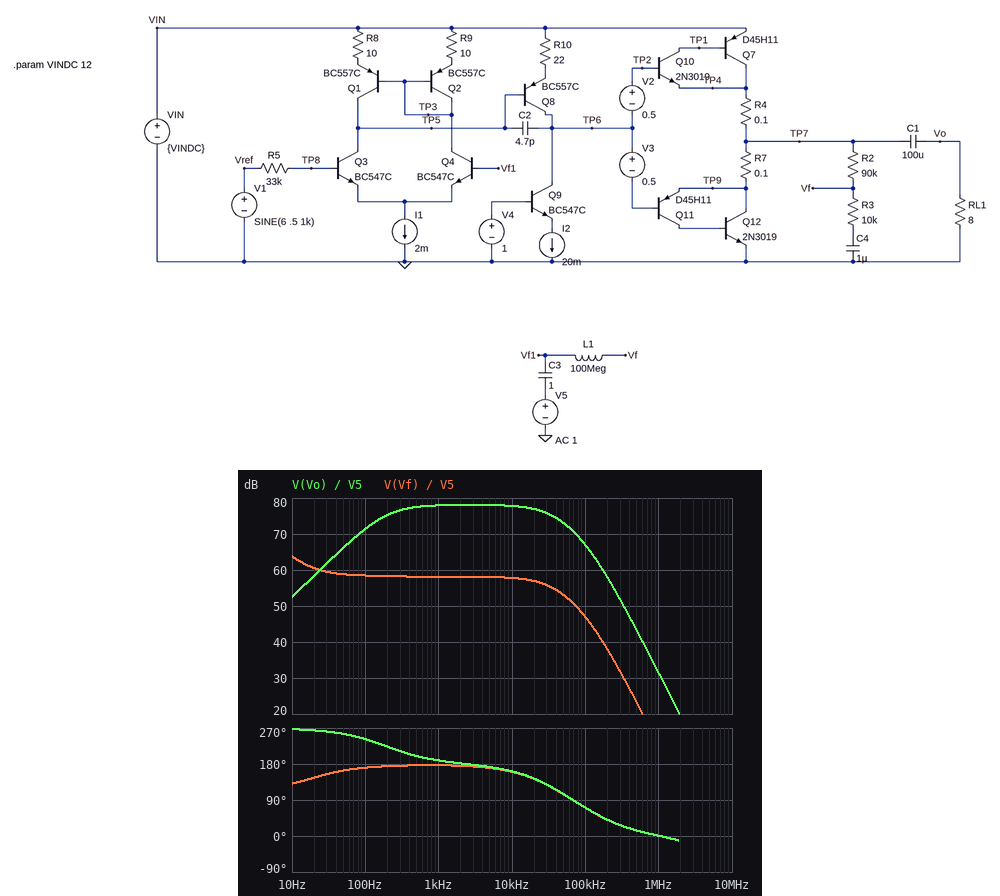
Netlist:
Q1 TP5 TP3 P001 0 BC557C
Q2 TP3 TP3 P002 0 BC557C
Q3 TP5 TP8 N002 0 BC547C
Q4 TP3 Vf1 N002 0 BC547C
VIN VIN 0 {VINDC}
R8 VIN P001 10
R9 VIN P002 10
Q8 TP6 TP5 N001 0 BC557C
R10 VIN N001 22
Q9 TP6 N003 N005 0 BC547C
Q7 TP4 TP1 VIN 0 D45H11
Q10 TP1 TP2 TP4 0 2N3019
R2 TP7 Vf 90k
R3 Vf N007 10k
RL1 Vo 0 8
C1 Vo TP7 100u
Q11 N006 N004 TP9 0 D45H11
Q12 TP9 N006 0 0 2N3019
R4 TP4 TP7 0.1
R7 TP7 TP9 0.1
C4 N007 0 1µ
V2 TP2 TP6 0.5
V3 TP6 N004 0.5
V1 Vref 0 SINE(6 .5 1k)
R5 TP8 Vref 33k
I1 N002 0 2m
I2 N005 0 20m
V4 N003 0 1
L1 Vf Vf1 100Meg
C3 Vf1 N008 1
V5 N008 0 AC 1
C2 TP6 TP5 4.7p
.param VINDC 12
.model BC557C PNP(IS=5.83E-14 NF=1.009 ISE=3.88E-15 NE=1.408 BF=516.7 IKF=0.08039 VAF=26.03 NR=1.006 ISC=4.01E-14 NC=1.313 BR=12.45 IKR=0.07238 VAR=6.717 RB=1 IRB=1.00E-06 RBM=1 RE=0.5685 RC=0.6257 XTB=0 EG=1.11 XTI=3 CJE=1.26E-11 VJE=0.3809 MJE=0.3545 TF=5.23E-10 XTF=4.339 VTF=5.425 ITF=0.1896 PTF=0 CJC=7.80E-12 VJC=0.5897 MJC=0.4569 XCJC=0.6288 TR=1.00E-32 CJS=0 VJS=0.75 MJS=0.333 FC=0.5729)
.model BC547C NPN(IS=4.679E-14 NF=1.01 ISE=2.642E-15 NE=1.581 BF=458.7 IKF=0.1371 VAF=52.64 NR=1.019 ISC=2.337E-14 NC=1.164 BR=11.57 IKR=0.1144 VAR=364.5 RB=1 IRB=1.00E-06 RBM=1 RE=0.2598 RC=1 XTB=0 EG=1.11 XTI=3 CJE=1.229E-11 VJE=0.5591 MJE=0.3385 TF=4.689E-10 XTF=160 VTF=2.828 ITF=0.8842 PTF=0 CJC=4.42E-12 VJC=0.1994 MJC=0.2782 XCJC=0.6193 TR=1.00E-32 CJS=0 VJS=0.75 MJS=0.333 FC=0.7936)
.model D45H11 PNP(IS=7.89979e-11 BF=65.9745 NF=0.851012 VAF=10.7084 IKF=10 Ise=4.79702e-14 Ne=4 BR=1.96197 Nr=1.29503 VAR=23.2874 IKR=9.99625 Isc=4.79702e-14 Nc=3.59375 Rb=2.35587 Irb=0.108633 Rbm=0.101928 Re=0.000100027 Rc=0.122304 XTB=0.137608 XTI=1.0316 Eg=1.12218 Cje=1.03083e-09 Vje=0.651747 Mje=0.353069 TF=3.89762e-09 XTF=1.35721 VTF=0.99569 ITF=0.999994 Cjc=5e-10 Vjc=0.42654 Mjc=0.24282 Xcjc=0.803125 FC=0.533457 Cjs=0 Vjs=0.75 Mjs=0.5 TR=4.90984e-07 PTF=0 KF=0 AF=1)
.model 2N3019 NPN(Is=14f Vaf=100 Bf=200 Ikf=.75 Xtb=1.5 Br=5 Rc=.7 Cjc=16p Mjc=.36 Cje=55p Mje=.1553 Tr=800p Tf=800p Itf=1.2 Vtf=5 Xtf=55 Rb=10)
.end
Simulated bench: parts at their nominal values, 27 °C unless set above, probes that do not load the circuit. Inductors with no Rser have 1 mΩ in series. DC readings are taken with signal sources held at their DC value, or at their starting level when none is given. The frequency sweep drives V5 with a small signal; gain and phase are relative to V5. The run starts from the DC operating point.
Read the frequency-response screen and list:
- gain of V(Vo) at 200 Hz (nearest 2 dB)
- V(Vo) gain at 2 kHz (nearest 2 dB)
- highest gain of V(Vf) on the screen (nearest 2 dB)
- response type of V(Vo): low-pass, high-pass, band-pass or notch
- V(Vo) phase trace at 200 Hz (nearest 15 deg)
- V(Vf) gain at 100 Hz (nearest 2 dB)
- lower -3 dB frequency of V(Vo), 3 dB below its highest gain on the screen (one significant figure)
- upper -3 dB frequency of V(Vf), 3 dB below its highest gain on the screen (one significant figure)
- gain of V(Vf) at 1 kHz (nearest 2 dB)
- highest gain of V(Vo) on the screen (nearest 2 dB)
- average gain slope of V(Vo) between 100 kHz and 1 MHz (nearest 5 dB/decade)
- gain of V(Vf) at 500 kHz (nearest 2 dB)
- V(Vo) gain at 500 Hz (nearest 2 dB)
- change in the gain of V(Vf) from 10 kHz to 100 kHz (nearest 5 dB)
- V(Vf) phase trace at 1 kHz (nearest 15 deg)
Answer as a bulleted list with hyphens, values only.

- 76 dB
- 78 dB
- 64 dB
- band-pass
- 225 deg
- 58 dB
- 200 Hz
- 20 Hz
- 58 dB
- 78 dB
- -35 dB/decade
- 24 dB
- 78 dB
- -10 dB
- 180 deg
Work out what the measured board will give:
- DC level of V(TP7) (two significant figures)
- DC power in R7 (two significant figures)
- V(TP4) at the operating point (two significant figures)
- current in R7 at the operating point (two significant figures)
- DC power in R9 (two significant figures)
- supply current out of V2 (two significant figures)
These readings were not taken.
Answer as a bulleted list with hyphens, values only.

- 6.1 V
- 900 µW
- 6.1 V
- 95 mA
- 9.4 µW
- 4.6 µA
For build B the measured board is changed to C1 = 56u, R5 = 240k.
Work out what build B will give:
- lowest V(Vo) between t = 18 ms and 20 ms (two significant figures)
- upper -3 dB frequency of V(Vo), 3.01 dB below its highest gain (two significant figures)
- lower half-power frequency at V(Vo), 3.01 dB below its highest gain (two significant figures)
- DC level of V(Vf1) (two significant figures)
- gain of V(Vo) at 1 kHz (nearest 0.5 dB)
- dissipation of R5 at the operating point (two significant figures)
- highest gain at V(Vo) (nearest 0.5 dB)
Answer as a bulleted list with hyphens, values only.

- -7.6 V
- 33 kHz
- 340 Hz
- 5.5 V
- 65.0 dB
- 1.0 µW
- 65.5 dB
